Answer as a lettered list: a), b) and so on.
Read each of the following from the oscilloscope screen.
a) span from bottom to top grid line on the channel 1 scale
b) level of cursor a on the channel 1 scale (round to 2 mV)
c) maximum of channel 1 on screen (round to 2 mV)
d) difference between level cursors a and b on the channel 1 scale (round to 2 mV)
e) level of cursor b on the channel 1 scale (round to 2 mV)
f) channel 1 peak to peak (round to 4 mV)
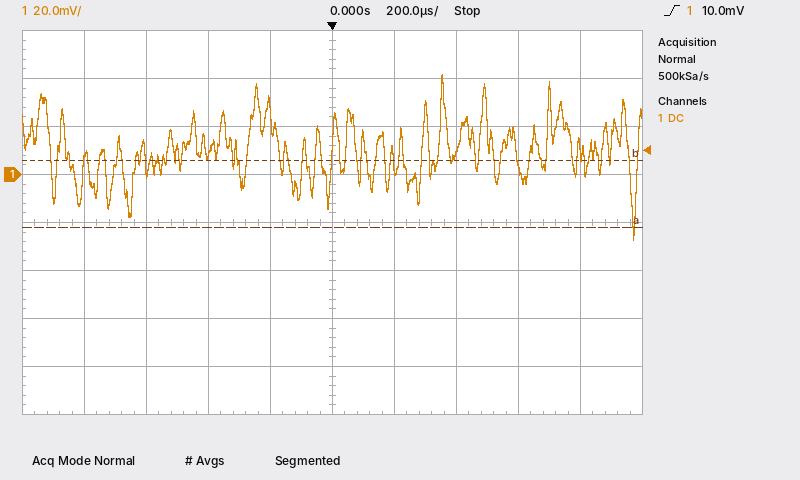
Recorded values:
a) 160 mV
b) -22 mV
c) 42 mV
d) 28 mV
e) 6 mV
f) 68 mV
